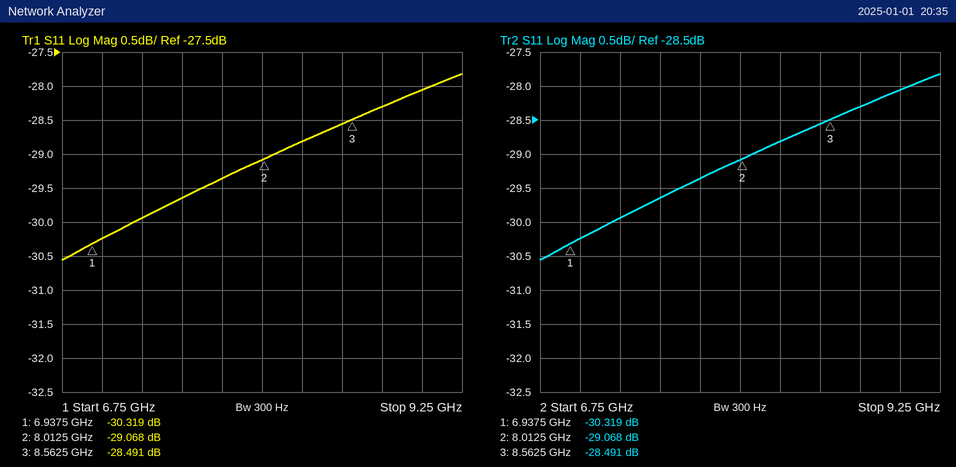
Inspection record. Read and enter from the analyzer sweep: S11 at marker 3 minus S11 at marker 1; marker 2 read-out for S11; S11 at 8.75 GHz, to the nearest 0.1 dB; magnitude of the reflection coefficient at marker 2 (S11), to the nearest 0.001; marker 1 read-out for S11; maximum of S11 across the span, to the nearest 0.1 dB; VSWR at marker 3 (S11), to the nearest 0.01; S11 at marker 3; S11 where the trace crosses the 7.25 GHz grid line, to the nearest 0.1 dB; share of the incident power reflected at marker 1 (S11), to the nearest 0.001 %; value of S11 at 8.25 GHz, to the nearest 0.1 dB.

1.828 dB
-29.068 dB
-28.3 dB
0.035
-30.319 dB
-27.8 dB
1.08
-28.491 dB
-29.9 dB
0.093 %
-28.8 dB
